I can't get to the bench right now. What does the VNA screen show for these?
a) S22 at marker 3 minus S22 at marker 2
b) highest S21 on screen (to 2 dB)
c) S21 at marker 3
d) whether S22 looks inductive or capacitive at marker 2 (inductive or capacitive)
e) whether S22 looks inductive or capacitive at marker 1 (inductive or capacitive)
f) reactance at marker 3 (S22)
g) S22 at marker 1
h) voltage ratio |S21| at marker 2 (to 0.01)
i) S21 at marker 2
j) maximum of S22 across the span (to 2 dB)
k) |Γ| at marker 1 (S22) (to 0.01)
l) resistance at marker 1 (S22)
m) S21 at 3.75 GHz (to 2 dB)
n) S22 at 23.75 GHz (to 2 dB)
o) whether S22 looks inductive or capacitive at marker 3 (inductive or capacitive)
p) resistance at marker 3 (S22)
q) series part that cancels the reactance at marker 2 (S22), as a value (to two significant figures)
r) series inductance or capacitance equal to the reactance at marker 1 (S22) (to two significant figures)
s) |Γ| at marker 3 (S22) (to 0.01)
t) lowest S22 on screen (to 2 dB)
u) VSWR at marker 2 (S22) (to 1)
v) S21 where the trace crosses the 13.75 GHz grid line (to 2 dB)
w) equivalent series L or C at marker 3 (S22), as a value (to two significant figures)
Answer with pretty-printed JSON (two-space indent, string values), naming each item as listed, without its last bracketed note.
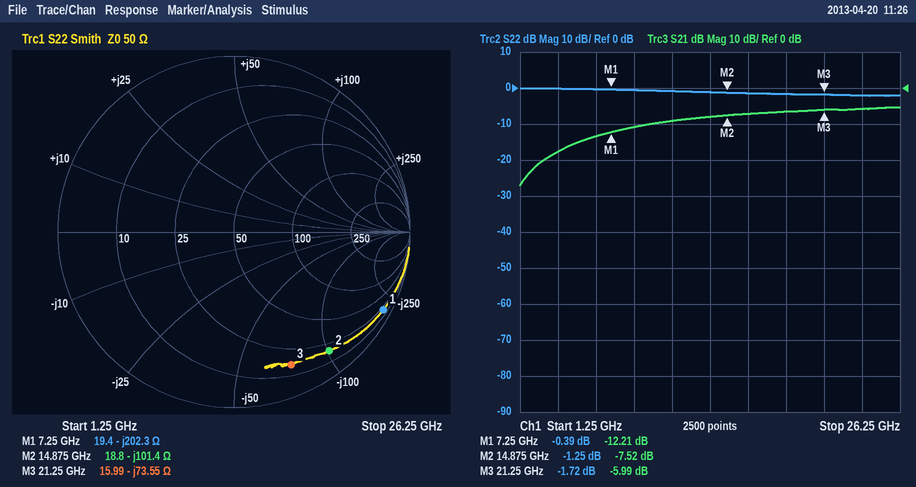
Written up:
{
  "S22 at marker 3 minus S22 at marker 2": "-0.47 dB",
  "highest S21 on screen": "-6 dB",
  "S21 at marker 3": "-5.99 dB",
  "whether S22 looks inductive or capacitive at marker 2": "capacitive",
  "whether S22 looks inductive or capacitive at marker 1": "capacitive",
  "reactance at marker 3": "-73.55 Ω",
  "S22 at marker 1": "-0.39 dB",
  "voltage ratio |S21| at marker 2": "0.42",
  "S21 at marker 2": "-7.52 dB",
  "maximum of S22 across the span": "0 dB",
  "|Γ| at marker 1 (S22)": "0.96",
  "resistance at marker 1": "19.4 Ω",
  "S21 at 3.75 GHz": "-18 dB",
  "S22 at 23.75 GHz": "-2 dB",
  "whether S22 looks inductive or capacitive at marker 3": "capacitive",
  "resistance at marker 3": "15.99 Ω",
  "series part that cancels the reactance at marker 2 (S22), as a value": "1.1 nH",
  "series inductance or capacitance equal to the reactance at marker 1 (S22)": "110 fF",
  "|Γ| at marker 3 (S22)": "0.82",
  "lowest S22 on screen": "-2 dB",
  "VSWR at marker 2 (S22)": "14",
  "S21 where the trace crosses the 13.75 GHz grid line": "-8 dB",
  "equivalent series L or C at marker 3 (S22), as a value": "100 fF"
}
